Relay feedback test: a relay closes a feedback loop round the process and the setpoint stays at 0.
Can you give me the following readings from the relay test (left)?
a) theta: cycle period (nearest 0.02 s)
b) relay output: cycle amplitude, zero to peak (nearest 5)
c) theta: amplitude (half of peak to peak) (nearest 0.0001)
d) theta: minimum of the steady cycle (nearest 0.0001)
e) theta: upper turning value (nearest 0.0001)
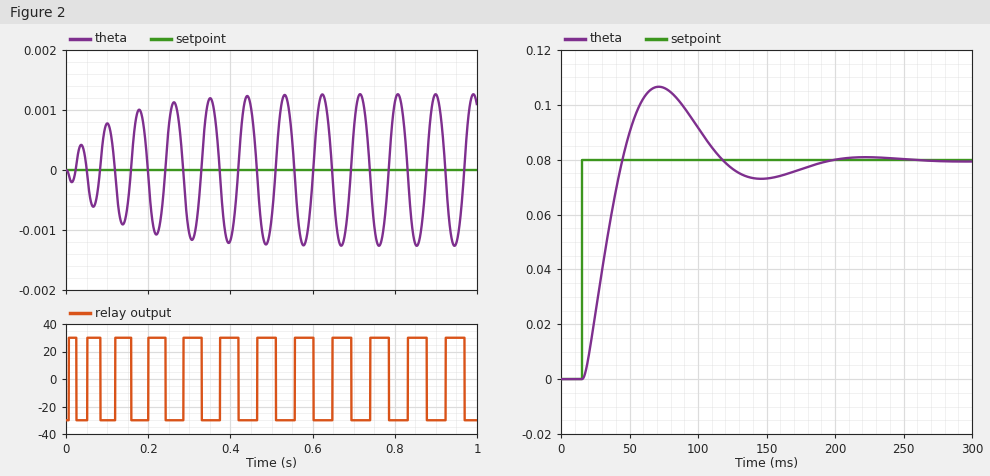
0.10 s
30
0.0013
-0.0013
0.0013
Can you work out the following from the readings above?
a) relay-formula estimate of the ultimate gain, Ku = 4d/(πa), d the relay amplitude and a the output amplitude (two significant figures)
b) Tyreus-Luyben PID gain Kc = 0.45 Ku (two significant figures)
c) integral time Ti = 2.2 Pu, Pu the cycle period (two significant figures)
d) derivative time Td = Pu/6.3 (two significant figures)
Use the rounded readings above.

29000
13000
0.22 s
0.016 s
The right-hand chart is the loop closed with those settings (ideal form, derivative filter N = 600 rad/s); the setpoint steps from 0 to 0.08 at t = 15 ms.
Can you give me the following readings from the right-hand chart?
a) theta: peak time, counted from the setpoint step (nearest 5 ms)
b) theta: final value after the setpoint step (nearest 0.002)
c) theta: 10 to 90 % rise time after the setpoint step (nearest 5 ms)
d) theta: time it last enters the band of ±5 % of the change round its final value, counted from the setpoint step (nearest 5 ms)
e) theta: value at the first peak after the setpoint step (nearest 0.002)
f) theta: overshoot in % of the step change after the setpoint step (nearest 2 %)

55 ms
0.080
20 ms
155 ms
0.106
34 %
